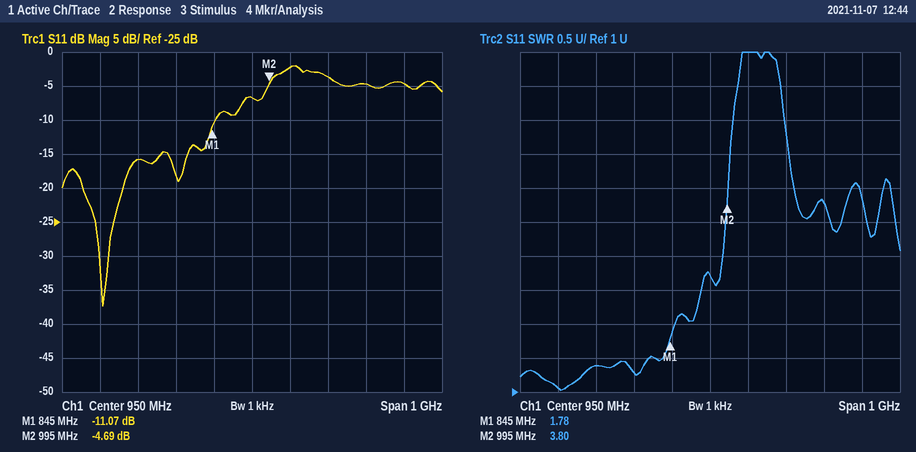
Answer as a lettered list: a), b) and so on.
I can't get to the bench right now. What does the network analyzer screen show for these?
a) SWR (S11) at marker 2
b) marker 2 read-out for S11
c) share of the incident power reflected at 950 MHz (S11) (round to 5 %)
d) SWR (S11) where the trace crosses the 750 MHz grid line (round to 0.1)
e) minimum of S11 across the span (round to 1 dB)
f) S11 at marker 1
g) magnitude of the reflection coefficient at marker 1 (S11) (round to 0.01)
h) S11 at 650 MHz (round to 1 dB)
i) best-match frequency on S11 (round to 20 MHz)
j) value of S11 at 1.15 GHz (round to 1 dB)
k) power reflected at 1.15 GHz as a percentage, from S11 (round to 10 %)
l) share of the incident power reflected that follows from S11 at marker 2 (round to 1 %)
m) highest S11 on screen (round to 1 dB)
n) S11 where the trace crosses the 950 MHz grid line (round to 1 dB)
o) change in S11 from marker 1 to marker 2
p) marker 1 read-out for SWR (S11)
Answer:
a) 3.80
b) -4.69 dB
c) 20 %
d) 1.3
e) -37 dB
f) -11.07 dB
g) 0.28
h) -16 dB
i) 560 MHz
j) -4 dB
k) 40 %
l) 34 %
m) -2 dB
n) -7 dB
o) 6.38 dB
p) 1.78
